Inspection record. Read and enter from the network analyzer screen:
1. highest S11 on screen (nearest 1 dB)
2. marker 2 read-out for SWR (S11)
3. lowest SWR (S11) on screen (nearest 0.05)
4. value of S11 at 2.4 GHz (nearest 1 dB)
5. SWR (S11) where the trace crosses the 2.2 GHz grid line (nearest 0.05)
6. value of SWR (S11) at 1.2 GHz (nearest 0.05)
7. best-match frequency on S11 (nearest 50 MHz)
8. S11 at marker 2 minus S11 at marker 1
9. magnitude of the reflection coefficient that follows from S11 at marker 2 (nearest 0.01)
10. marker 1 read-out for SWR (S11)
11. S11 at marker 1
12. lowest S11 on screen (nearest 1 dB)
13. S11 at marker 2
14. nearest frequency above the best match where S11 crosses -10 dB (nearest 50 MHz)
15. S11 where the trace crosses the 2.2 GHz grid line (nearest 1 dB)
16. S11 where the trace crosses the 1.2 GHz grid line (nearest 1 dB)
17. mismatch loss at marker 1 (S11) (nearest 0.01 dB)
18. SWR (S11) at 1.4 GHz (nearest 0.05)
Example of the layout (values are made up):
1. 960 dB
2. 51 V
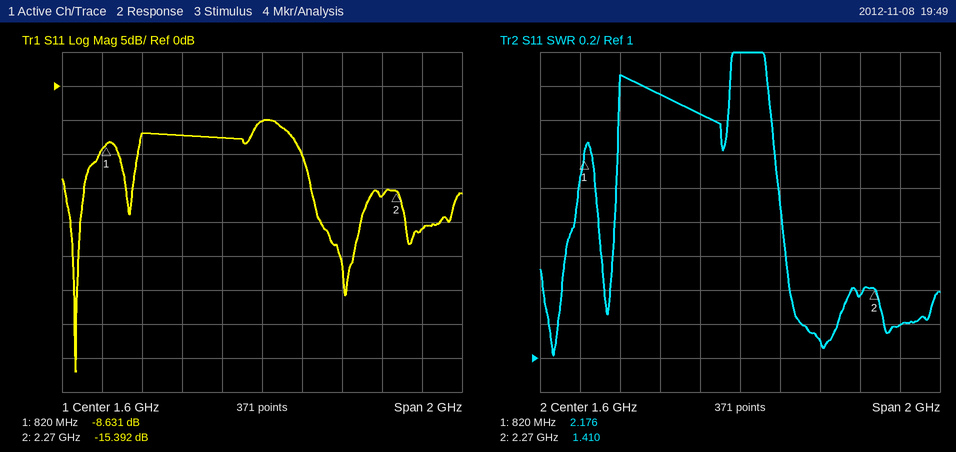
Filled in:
1. -5 dB
2. 1.410
3. 1.00
4. -21 dB
5. 1.35
6. 2.55
7. 650 MHz
8. -6.761 dB
9. 0.17
10. 2.176
11. -8.631 dB
12. -42 dB
13. -15.392 dB
14. 800 MHz
15. -16 dB
16. -7 dB
17. 0.64 dB
18. 2.45
